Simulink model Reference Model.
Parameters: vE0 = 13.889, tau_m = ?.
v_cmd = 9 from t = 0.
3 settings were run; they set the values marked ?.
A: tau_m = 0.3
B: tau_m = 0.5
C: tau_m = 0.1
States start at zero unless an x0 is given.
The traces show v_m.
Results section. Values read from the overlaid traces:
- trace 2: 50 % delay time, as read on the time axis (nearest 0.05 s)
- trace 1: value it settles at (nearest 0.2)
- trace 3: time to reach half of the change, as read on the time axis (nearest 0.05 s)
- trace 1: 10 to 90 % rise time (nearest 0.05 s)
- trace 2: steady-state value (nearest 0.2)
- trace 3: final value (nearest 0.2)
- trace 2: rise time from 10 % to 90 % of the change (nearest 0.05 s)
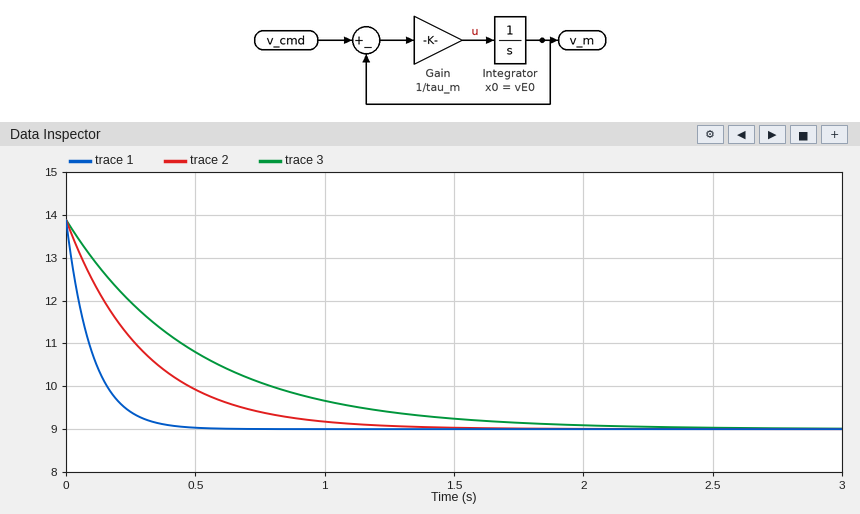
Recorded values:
0.20 s
9.0
0.35 s
0.20 s
9.0
9.0
0.65 s
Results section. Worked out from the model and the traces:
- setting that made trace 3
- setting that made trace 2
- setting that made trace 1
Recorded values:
B
A
C
